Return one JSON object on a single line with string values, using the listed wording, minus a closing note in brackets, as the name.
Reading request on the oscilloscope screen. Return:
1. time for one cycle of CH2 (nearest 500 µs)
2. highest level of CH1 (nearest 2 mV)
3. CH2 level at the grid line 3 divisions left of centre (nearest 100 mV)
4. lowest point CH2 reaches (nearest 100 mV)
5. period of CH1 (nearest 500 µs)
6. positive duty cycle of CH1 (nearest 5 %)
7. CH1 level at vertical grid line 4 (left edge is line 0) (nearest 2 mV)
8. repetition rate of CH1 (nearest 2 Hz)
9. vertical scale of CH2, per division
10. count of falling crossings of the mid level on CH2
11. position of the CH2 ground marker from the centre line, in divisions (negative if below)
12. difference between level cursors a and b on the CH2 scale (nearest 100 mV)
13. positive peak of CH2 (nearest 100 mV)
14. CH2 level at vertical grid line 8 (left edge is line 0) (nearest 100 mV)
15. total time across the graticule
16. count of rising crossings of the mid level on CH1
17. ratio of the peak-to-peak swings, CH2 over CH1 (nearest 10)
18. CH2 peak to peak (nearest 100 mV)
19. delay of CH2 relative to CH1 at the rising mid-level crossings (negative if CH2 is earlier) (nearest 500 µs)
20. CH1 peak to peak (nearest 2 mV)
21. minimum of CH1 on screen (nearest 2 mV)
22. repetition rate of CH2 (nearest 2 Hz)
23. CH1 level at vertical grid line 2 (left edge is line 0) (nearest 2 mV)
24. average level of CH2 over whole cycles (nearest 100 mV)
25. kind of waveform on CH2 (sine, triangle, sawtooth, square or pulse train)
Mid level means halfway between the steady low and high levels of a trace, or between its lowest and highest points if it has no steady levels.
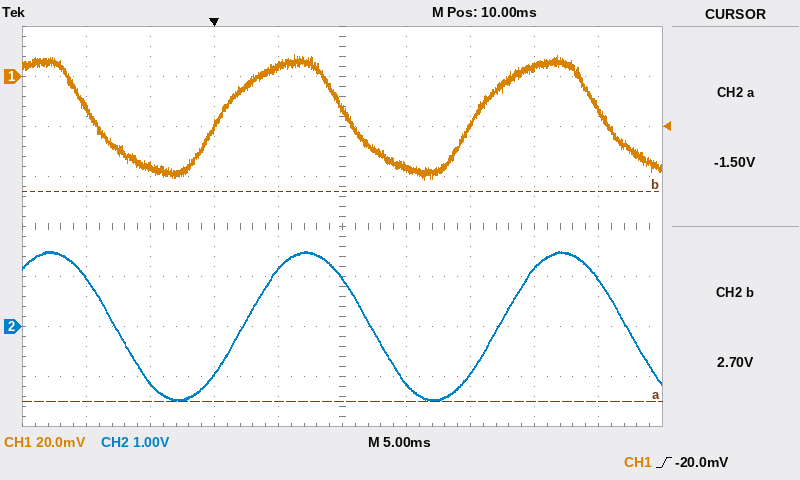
{"time for one cycle of CH2": "20.0 ms", "highest level of CH1": "8 mV", "CH2 level at the grid line 3 divisions left of centre": "-1.1 V", "lowest point CH2 reaches": "-1.5 V", "period of CH1": "20.0 ms", "positive duty cycle of CH1": "50 %", "CH1 level at vertical grid line 4 (left edge is line 0)": "4 mV", "repetition rate of CH1": "50 Hz", "vertical scale of CH2, per division": "1 V", "count of falling crossings of the mid level on CH2": "3", "position of the CH2 ground marker from the centre line, in divisions": "-2.0 div", "difference between level cursors a and b on the CH2 scale": "4.2 V", "positive peak of CH2": "1.5 V", "CH2 level at vertical grid line 8 (left edge is line 0)": "1.2 V", "total time across the graticule": "50 ms", "count of rising crossings of the mid level on CH1": "2", "ratio of the peak-to-peak swings, CH2 over CH1": "60", "CH2 peak to peak": "3.0 V", "delay of CH2 relative to CH1 at the rising mid-level crossings (negative if CH2 is earlier)": "+2.0 ms", "CH1 peak to peak": "50 mV", "minimum of CH1 on screen": "-42 mV", "repetition rate of CH2": "50 Hz", "CH1 level at vertical grid line 2 (left edge is line 0)": "-36 mV", "average level of CH2 over whole cycles": "0.0 V", "kind of waveform on CH2": "sine"}
